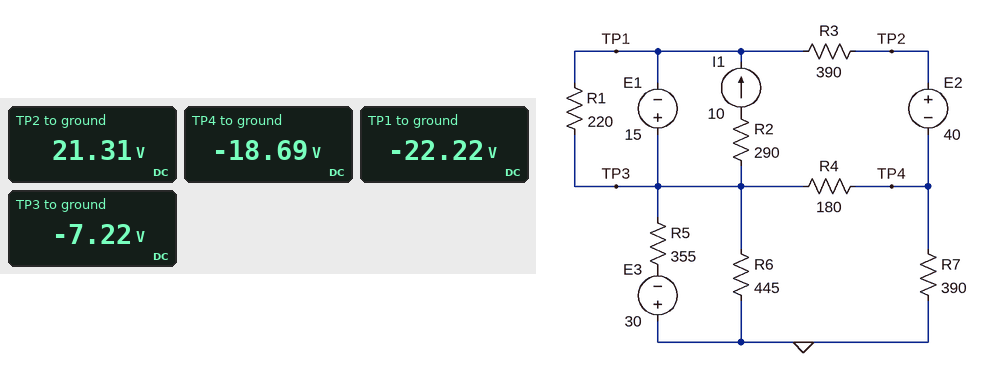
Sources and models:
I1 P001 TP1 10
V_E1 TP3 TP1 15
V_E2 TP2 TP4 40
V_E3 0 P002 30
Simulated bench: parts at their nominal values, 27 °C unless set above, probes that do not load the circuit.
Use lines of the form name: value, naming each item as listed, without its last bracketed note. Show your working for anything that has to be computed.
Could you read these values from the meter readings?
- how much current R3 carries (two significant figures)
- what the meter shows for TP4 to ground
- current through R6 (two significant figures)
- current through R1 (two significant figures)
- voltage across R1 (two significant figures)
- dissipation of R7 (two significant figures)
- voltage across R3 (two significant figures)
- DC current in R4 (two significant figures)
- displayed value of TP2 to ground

how much current R3 carries: (21.31 V - (-22.22 V)) / 390 Ω = 110 mA
what the meter shows for TP4 to ground: -18.69 V
current through R6: (0 V - (-7.22 V)) / 445 Ω = 16 mA
current through R1: (-7.22 V - (-22.22 V)) / 220 Ω = 68 mA
voltage across R1: -7.22 V - (-22.22 V) = 15 V
dissipation of R7: (0 V - (-18.69 V))^2 / 390 Ω = 900 mW
voltage across R3: 21.31 V - (-22.22 V) = 44 V
DC current in R4: (-7.22 V - (-18.69 V)) / 180 Ω = 64 mA
displayed value of TP2 to ground: 21.31 V
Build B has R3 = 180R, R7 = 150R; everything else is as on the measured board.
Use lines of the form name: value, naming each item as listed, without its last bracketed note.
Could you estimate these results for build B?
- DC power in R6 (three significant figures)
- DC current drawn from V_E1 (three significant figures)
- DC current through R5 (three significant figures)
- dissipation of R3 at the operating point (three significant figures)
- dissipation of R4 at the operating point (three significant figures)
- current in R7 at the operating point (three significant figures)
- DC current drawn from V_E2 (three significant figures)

DC power in R6: 23.9 mW
DC current drawn from V_E1: 10.3 A
DC current through R5: 93.7 mA
dissipation of R3 at the operating point: 7.44 W
dissipation of R4 at the operating point: 1.88 W
current in R7 at the operating point: 101 mA
DC current drawn from V_E2: 203 mA
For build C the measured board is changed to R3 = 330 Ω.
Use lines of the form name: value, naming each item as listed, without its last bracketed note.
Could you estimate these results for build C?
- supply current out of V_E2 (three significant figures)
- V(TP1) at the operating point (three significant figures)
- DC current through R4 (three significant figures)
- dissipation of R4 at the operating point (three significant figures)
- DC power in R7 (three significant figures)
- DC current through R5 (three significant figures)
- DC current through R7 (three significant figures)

supply current out of V_E2: 126 mA
V(TP1) at the operating point: -21.6 V
DC current through R4: 74.7 mA
dissipation of R4 at the operating point: 1.00 W
DC power in R7: 1.03 W
DC current through R5: 66.0 mA
DC current through R7: 51.3 mA
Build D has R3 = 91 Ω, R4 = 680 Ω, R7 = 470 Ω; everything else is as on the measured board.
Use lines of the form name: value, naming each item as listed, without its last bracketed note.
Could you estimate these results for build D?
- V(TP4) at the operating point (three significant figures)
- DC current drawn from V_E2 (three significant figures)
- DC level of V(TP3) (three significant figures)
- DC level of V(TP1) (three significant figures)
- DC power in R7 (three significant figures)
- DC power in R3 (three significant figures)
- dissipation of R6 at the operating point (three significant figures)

V(TP4) at the operating point: -41.0 V
DC current drawn from V_E2: 148 mA
DC level of V(TP3): 530 mV
DC level of V(TP1): -14.5 V
DC power in R7: 3.57 W
DC power in R3: 2.00 W
dissipation of R6 at the operating point: 632 µW
